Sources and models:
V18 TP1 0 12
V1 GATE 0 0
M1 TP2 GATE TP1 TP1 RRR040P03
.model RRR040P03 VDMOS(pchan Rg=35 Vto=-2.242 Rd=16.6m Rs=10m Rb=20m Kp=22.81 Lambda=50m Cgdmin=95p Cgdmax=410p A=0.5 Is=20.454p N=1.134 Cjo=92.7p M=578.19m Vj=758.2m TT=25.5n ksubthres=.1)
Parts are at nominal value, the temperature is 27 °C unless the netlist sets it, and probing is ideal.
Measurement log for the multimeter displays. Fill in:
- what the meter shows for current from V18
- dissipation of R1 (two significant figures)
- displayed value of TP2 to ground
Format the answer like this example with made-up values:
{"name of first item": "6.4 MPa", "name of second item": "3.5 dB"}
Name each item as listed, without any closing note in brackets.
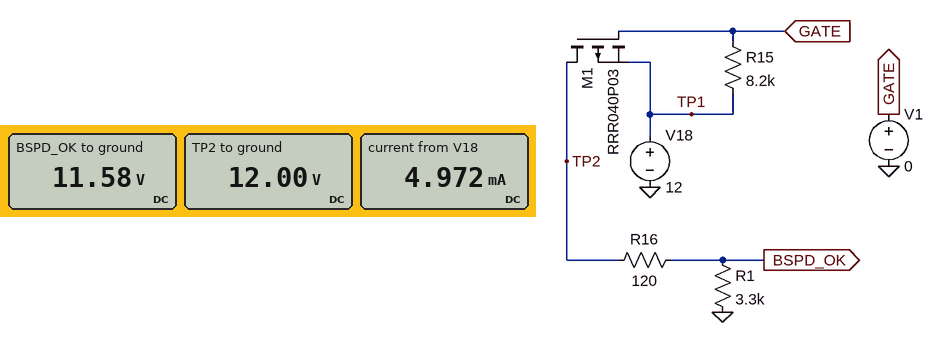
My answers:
{"what the meter shows for current from V18": "4.972 mA", "dissipation of R1": "41 mW", "displayed value of TP2 to ground": "12.00 V"}
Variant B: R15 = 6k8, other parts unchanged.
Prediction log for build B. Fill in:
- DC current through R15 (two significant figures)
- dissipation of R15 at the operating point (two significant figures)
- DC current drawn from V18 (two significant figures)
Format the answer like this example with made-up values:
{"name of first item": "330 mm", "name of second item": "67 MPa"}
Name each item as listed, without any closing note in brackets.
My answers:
{"DC current through R15": "1.8 mA", "dissipation of R15 at the operating point": "21 mW", "DC current drawn from V18": "5.3 mA"}
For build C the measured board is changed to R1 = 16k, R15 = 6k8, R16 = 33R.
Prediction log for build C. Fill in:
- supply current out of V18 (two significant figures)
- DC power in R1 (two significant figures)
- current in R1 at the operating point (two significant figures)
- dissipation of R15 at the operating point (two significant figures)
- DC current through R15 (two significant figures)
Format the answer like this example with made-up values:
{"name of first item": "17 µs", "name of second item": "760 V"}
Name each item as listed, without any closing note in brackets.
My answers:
{"supply current out of V18": "2.5 mA", "DC power in R1": "9.0 mW", "current in R1 at the operating point": "750 µA", "dissipation of R15 at the operating point": "21 mW", "DC current through R15": "1.8 mA"}
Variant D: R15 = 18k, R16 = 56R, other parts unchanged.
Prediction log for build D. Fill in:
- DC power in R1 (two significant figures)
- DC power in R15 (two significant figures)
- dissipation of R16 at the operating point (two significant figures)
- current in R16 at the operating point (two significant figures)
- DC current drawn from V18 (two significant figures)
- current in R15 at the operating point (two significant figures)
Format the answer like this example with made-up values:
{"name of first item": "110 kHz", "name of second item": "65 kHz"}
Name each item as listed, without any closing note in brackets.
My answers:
{"DC power in R1": "42 mW", "DC power in R15": "8.0 mW", "dissipation of R16 at the operating point": "720 µW", "current in R16 at the operating point": "3.6 mA", "DC current drawn from V18": "4.2 mA", "current in R15 at the operating point": "670 µA"}
